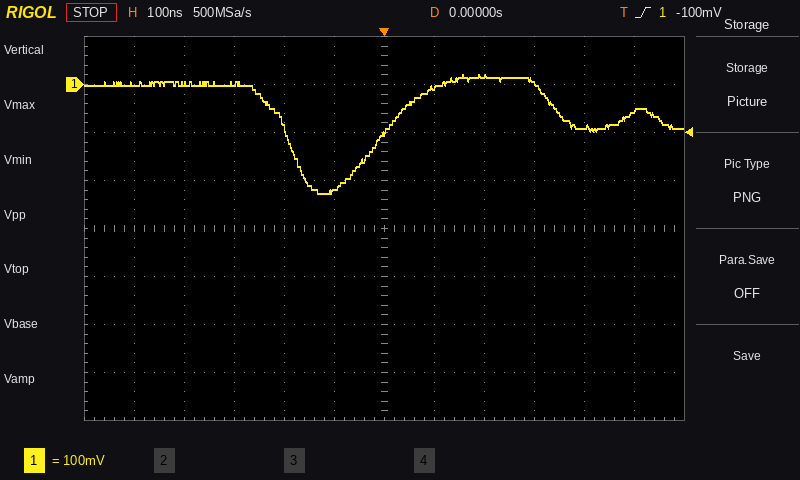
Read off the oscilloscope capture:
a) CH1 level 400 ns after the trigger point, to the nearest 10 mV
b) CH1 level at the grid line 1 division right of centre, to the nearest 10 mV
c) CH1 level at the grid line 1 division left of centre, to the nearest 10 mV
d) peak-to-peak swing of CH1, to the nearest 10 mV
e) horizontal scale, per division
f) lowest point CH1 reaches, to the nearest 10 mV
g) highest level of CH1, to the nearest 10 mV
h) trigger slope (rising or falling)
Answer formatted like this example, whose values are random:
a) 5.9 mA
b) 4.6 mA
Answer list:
a) -90 mV
b) -10 mV
c) -220 mV
d) 250 mV
e) 100 ns
f) -230 mV
g) 20 mV
h) rising
